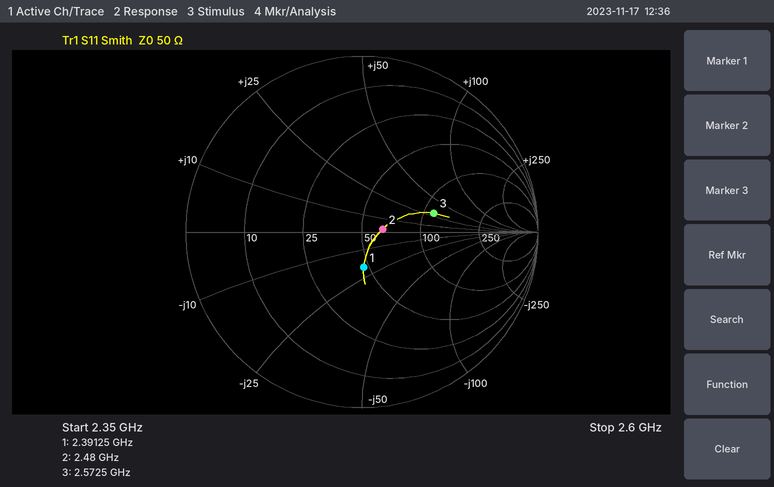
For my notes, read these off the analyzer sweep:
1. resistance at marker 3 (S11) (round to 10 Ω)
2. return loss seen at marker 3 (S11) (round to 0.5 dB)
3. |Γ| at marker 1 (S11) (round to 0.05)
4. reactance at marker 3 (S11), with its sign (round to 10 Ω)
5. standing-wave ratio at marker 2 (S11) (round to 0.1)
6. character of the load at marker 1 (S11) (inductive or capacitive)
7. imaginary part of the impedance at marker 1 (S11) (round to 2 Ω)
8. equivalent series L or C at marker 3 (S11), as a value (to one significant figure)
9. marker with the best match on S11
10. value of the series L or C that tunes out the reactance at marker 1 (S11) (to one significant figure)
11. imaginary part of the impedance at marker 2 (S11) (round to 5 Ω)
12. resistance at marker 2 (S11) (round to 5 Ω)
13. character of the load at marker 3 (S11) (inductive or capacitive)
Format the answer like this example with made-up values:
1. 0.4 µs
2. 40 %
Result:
1. 110 Ω
2. 7.5 dB
3. 0.20
4. +30 Ω
5. 1.3
6. capacitive
7. -20 Ω
8. 2 nH
9. marker 2
10. 1 nH
11. 0 Ω
12. 65 Ω
13. inductive
